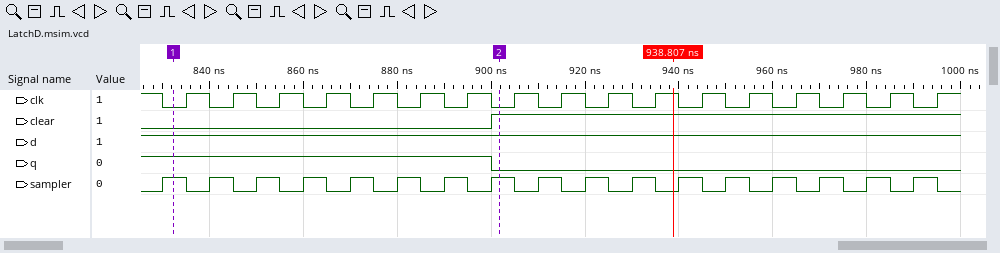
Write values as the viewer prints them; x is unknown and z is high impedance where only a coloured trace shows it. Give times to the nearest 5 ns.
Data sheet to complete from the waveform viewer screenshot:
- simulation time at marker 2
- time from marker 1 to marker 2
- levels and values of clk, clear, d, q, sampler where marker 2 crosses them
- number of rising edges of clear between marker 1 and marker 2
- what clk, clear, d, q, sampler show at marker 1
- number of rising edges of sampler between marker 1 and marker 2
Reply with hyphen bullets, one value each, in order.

- 900 ns
- 70 ns
- clk=0, clear=1, d=1, q=0, sampler=1
- 1
- clk=0, clear=0, d=1, q=1, sampler=1
- 7
